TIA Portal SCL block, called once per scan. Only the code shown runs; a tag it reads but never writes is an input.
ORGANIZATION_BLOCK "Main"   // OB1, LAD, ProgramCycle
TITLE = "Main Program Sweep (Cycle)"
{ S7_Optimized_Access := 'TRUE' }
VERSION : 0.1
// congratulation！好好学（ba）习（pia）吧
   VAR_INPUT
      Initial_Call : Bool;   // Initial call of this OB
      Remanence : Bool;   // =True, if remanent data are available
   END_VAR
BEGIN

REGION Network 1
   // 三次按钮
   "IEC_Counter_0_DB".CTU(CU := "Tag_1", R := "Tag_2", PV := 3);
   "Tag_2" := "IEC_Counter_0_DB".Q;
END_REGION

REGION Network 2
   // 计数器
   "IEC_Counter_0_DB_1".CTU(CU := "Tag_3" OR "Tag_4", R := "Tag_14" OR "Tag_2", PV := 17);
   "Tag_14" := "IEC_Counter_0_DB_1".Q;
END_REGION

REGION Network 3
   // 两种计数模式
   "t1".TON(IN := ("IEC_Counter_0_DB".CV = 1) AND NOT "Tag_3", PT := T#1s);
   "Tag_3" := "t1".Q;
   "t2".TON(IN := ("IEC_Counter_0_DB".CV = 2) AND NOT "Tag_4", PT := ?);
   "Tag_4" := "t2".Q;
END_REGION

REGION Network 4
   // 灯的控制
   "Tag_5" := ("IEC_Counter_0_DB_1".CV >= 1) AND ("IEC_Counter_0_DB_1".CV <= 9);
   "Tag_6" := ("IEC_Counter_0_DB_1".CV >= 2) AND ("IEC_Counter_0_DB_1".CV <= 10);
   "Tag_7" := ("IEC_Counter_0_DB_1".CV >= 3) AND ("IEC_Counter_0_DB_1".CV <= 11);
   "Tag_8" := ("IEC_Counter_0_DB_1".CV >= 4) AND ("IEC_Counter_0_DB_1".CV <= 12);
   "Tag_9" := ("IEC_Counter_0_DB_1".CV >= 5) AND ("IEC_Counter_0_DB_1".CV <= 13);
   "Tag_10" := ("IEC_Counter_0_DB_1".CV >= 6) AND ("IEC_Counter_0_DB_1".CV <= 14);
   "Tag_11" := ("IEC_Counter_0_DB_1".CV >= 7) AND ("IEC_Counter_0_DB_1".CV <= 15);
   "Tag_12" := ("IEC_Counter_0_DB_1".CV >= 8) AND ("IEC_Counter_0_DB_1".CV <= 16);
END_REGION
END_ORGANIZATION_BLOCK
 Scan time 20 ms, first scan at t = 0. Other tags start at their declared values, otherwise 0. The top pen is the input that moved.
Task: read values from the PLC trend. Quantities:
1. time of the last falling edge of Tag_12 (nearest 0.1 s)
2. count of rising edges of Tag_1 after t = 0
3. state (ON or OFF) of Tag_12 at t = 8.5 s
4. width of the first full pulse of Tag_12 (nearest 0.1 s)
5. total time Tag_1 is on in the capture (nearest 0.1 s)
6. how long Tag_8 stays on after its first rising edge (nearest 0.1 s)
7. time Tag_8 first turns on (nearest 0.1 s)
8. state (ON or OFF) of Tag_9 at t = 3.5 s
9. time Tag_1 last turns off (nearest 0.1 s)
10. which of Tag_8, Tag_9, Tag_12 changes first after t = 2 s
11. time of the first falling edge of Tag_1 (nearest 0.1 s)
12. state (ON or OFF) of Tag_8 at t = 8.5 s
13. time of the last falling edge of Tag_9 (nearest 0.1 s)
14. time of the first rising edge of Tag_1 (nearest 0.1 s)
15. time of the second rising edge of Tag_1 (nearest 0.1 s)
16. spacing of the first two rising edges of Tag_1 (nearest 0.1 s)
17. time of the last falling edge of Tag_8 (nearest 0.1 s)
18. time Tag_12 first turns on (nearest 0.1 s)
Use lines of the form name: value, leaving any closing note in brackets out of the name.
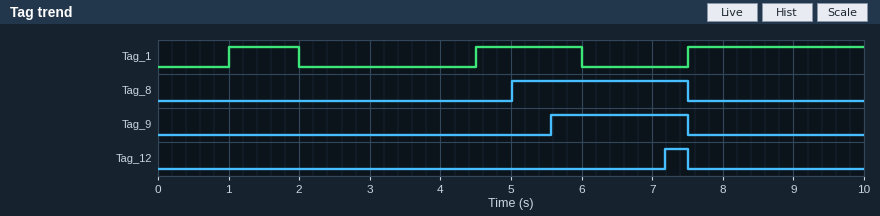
time of the last falling edge of Tag_12: 7.5 s
count of rising edges of Tag_1 after t = 0: 3
state (ON or OFF) of Tag_12 at t = 8.5 s: OFF
width of the first full pulse of Tag_12: 0.3 s
total time Tag_1 is on in the capture: 5.0 s
how long Tag_8 stays on after its first rising edge: 2.5 s
time Tag_8 first turns on: 5.0 s
state (ON or OFF) of Tag_9 at t = 3.5 s: OFF
time Tag_1 last turns off: 6.0 s
which of Tag_8, Tag_9, Tag_12 changes first after t = 2 s: Tag_8
time of the first falling edge of Tag_1: 2.0 s
state (ON or OFF) of Tag_8 at t = 8.5 s: OFF
time of the last falling edge of Tag_9: 7.5 s
time of the first rising edge of Tag_1: 1.0 s
time of the second rising edge of Tag_1: 4.5 s
spacing of the first two rising edges of Tag_1: 3.5 s
time of the last falling edge of Tag_8: 7.5 s
time Tag_12 first turns on: 7.2 s
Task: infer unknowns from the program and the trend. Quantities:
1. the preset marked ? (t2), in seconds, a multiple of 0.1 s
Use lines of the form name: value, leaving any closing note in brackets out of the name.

the preset marked ? (t2), in seconds, a multiple of 0.1 s: 0.5 s
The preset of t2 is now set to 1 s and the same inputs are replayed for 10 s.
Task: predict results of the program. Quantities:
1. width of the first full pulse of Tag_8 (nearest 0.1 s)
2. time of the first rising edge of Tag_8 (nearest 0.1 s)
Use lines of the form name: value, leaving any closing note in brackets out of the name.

width of the first full pulse of Tag_8: 2.0 s
time of the first rising edge of Tag_8: 5.5 s
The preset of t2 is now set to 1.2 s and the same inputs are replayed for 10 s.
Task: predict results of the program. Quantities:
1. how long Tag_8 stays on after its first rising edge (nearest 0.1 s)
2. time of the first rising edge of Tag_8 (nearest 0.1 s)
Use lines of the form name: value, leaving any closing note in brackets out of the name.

how long Tag_8 stays on after its first rising edge: 1.8 s
time of the first rising edge of Tag_8: 5.7 s
